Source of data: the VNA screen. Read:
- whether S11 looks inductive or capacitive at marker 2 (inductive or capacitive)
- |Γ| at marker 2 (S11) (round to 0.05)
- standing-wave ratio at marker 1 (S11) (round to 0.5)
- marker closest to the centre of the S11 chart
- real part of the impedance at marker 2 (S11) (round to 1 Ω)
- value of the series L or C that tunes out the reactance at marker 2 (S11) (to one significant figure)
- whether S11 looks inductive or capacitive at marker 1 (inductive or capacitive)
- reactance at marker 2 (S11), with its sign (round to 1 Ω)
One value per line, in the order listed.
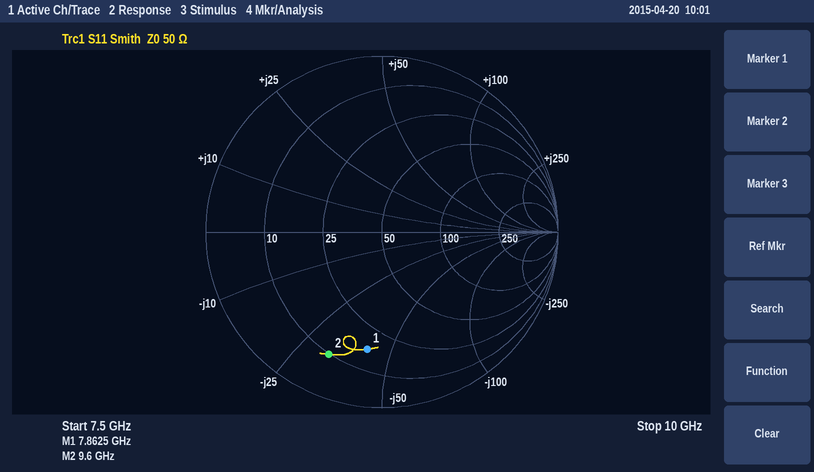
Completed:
capacitive
0.75
5.0
marker 1
10 Ω
500 pH
capacitive
-32 Ω
